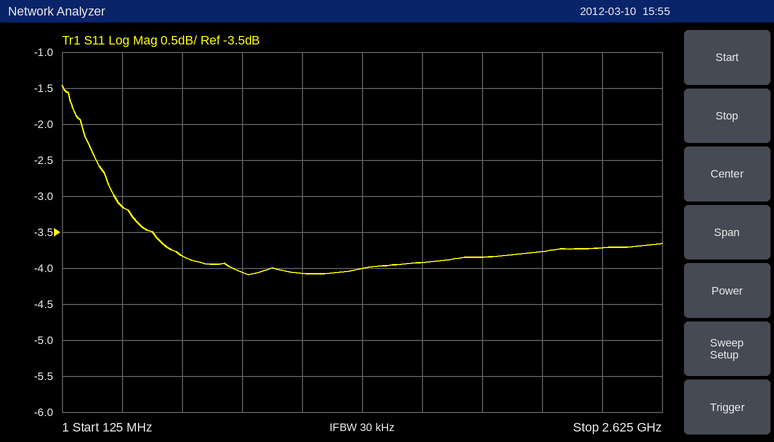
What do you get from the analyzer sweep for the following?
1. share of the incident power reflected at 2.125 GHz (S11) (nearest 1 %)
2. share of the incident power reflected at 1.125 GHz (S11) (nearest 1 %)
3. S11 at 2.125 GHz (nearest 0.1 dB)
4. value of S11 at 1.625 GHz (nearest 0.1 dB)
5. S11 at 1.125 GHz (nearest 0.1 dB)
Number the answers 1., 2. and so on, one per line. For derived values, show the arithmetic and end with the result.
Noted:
1. 10^(-3.8/10) ≈ 42 %
2. 10^(-4.1/10) ≈ 39 %
3. -3.8 dB
4. -3.9 dB
5. -4.1 dB
